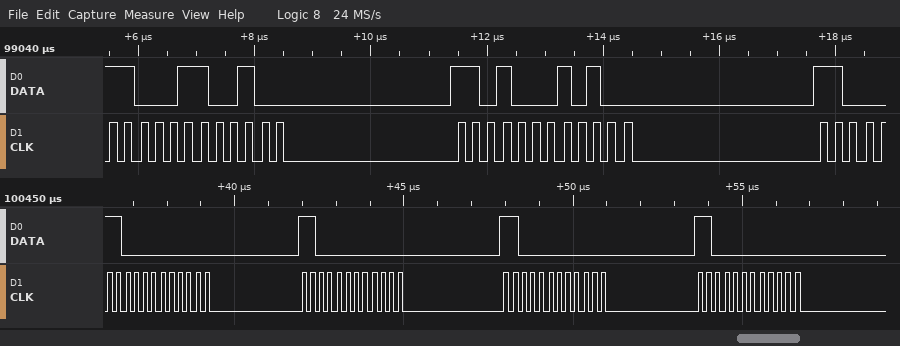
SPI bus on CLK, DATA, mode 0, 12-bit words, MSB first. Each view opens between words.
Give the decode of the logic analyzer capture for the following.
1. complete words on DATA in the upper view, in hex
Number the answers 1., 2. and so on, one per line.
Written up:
1. C64, D14
